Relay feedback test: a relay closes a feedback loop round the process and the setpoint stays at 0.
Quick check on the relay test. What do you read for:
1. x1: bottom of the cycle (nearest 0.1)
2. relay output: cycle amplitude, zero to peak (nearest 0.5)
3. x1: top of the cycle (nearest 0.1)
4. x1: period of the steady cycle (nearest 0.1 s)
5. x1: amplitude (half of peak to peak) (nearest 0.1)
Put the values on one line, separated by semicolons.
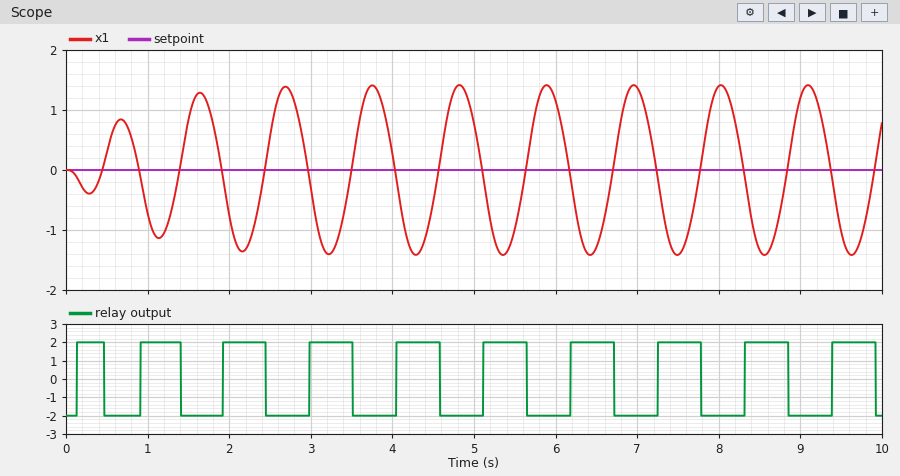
-1.4; 2.0; 1.4; 1.1 s; 1.4
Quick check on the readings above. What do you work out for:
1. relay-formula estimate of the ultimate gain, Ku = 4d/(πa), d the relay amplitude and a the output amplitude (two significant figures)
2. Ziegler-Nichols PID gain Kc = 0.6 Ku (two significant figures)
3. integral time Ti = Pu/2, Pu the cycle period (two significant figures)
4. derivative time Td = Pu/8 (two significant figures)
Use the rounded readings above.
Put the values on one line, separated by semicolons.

1.8; 1.1; 0.55 s; 0.14 s
